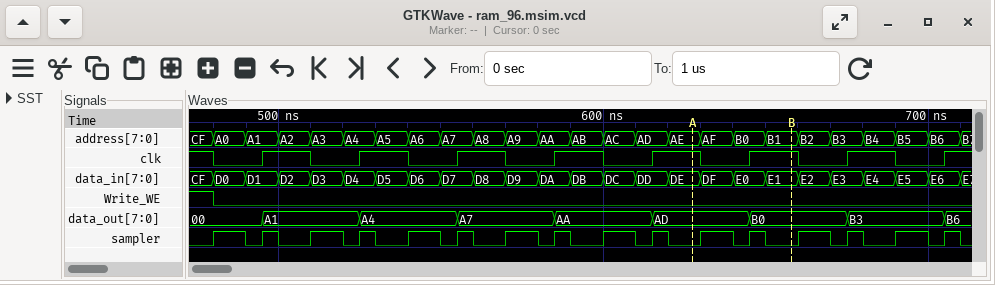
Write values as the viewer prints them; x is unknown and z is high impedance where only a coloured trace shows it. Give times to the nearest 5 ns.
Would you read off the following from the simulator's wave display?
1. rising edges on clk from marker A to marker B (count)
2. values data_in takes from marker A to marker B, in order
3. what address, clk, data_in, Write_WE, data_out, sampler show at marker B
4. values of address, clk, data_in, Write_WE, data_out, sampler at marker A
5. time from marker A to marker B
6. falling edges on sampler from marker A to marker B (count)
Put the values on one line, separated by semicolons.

1; DE, DF, E0, E1; address=B1, clk=1, data_in=E1, Write_WE=0, data_out=B0, sampler=0; address=AE, clk=1, data_in=DE, Write_WE=0, data_out=AD, sampler=0; 30 ns; 2
